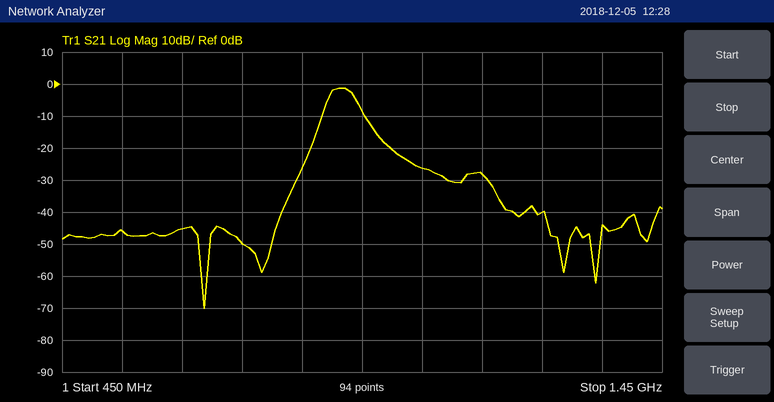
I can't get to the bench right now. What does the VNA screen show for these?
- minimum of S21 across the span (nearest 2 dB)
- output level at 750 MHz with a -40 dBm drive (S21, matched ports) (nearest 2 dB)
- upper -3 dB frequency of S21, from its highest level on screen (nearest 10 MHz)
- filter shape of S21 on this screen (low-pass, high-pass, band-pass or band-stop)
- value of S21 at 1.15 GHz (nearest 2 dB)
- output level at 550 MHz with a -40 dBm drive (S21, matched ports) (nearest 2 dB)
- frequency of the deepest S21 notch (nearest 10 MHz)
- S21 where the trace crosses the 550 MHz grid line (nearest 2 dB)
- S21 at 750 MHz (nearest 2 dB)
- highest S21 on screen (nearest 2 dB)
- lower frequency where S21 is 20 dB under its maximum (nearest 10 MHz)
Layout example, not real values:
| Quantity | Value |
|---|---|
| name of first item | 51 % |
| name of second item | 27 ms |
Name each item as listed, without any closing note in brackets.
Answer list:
| Quantity | Value |
|---|---|
| minimum of S21 across the span | -70 dB |
| output level at 750 MHz with a -40 dBm drive (S21, matched ports) | -90 dBm |
| upper -3 dB frequency of S21, from its highest level on screen | 940 MHz |
| filter shape of S21 on this screen | band-pass |
| value of S21 at 1.15 GHz | -28 dB |
| output level at 550 MHz with a -40 dBm drive (S21, matched ports) | -86 dBm |
| frequency of the deepest S21 notch | 690 MHz |
| S21 where the trace crosses the 550 MHz grid line | -46 dB |
| S21 at 750 MHz | -50 dB |
| highest S21 on screen | -2 dB |
| lower frequency where S21 is 20 dB under its maximum | 860 MHz |
